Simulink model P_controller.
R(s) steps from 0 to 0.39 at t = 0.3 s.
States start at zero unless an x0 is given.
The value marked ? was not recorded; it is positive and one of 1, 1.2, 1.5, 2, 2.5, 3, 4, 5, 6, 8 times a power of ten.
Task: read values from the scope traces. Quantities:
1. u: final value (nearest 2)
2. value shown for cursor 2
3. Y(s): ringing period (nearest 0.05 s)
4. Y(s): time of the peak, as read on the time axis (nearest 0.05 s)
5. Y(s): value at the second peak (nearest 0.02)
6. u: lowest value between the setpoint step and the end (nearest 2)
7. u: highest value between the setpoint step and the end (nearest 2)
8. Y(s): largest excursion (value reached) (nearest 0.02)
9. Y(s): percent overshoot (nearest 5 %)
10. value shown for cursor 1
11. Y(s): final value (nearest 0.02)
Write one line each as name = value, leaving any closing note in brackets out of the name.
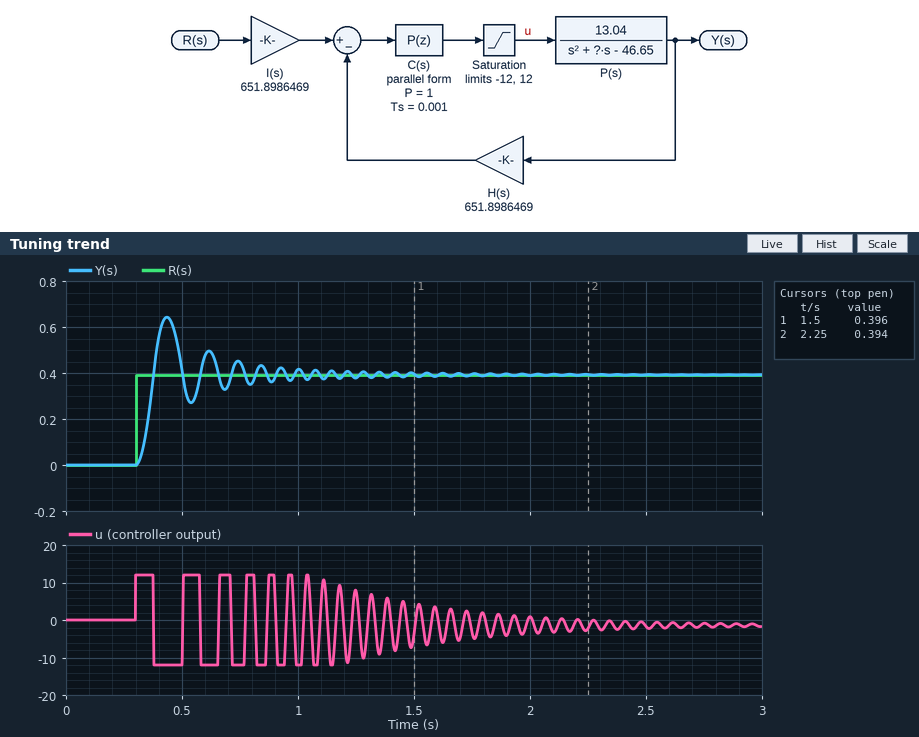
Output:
u: final value = -2
value shown for cursor 2 = 0.394
Y(s): ringing period = 0.20 s
Y(s): time of the peak, as read on the time axis = 0.45 s
Y(s): value at the second peak = 0.50
u: lowest value between the setpoint step and the end = -12
u: highest value between the setpoint step and the end = 12
Y(s): largest excursion (value reached) = 0.64
Y(s): percent overshoot = 65 %
value shown for cursor 1 = 0.396
Y(s): final value = 0.40
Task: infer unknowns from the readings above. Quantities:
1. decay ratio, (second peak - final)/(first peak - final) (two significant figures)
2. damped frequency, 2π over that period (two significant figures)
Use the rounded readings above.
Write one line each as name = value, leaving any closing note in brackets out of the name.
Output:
decay ratio, (second peak - final)/(first peak - final) = 0.42
damped frequency, 2π over that period = 31 rad/s
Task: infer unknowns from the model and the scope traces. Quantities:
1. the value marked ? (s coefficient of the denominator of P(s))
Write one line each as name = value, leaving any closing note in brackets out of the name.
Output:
the value marked ? (s coefficient of the denominator of P(s)) = 8
